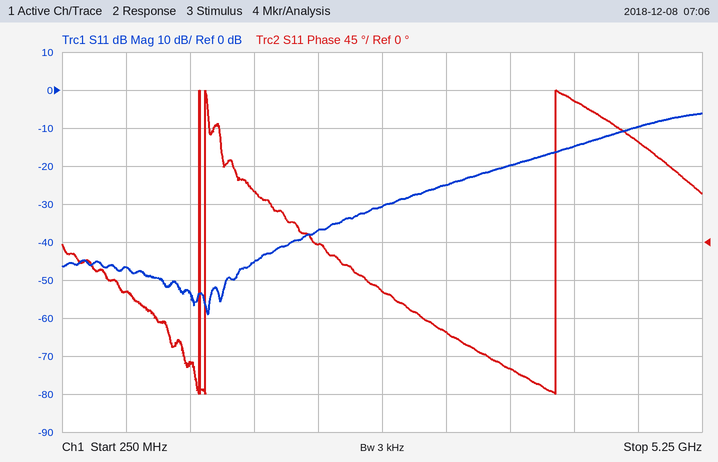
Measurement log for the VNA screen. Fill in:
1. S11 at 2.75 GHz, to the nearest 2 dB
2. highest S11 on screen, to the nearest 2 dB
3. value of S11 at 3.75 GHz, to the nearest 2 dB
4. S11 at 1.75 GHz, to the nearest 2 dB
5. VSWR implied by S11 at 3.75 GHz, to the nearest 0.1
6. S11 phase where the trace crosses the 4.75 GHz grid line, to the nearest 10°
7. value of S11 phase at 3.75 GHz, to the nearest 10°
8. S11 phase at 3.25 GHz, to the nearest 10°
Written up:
-30 dB
-6 dB
-20 dB
-46 dB
1.2
120°
-150°
-110°
